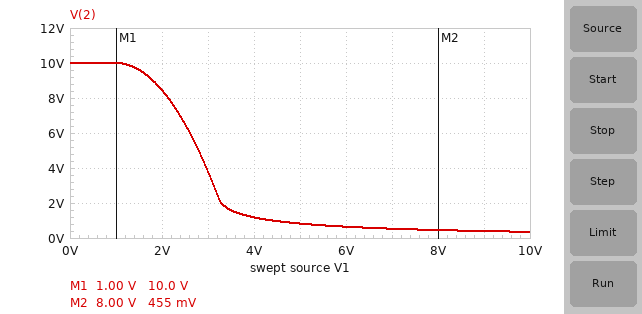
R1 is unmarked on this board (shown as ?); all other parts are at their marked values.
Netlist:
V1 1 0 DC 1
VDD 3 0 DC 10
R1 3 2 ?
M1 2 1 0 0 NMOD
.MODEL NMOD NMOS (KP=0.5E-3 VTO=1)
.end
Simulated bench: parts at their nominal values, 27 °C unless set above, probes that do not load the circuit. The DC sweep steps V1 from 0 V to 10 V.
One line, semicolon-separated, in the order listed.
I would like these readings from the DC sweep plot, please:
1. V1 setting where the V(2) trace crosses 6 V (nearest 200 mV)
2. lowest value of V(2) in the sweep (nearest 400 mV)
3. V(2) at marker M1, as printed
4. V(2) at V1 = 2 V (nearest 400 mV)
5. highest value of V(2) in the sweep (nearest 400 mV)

2.6 V; 400 mV; 10.0 V; 8.4 V; 10.0 V
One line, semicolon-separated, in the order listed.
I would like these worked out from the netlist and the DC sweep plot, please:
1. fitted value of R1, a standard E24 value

6.2 kΩ
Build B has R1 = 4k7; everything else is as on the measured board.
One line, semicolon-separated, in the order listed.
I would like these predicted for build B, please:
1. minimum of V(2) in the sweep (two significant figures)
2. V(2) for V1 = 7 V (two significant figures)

460 mV; 700 mV
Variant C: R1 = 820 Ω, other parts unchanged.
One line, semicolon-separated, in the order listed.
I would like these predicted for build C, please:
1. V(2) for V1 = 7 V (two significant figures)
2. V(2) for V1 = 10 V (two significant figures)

3.7 V; 2.4 V
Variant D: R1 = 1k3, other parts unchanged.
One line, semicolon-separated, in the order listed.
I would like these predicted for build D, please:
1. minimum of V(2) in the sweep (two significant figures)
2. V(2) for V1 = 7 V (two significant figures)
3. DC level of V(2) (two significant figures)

1.6 V; 2.4 V; 10 V
